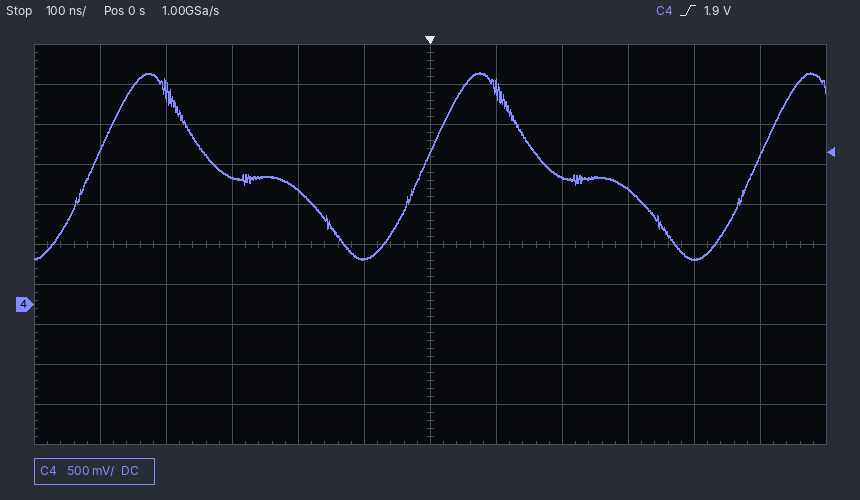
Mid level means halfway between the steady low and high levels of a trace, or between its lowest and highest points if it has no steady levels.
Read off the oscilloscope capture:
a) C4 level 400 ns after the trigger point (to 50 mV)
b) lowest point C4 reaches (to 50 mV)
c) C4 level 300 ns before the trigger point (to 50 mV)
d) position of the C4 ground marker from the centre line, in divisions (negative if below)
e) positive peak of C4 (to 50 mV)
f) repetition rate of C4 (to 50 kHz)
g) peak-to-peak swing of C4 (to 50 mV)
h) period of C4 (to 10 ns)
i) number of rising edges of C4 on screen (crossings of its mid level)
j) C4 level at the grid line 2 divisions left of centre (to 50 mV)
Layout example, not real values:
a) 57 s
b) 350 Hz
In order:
a) 550 mV
b) 550 mV
c) 1.60 V
d) -1.5 div
e) 2.90 V
f) 2.00 MHz
g) 2.35 V
h) 500 ns
i) 3
j) 1.45 V
